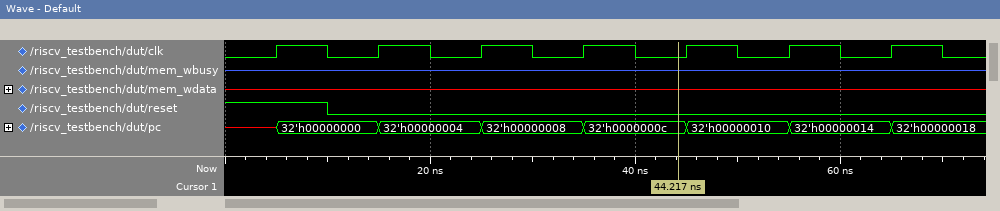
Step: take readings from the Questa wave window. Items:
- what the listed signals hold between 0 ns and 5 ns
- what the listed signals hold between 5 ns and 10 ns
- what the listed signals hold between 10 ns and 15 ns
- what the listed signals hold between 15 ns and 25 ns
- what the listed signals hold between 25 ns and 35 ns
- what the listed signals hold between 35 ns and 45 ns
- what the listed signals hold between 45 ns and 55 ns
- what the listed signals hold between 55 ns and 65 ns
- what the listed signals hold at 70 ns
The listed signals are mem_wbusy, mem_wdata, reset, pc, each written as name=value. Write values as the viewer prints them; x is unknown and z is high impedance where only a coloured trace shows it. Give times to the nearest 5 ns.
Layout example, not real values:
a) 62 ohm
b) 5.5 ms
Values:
a) mem_wbusy=z, mem_wdata=x, reset=1, pc=x
b) mem_wbusy=z, mem_wdata=x, reset=1, pc=32'h00000000
c) mem_wbusy=z, mem_wdata=x, reset=0, pc=32'h00000000
d) mem_wbusy=z, mem_wdata=x, reset=0, pc=32'h00000004
e) mem_wbusy=z, mem_wdata=x, reset=0, pc=32'h00000008
f) mem_wbusy=z, mem_wdata=x, reset=0, pc=32'h0000000c
g) mem_wbusy=z, mem_wdata=x, reset=0, pc=32'h00000010
h) mem_wbusy=z, mem_wdata=x, reset=0, pc=32'h00000014
i) mem_wbusy=z, mem_wdata=x, reset=0, pc=32'h00000018
